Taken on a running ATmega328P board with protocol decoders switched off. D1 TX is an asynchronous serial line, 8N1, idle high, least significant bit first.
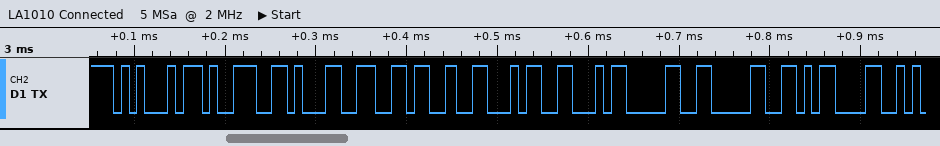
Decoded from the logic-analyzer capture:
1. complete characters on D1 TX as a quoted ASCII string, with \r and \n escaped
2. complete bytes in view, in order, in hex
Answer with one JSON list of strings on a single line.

["\"E916FF00\\r\"", "0x45 0x39 0x31 0x36 0x46 0x46 0x30 0x30 0x0D"]
